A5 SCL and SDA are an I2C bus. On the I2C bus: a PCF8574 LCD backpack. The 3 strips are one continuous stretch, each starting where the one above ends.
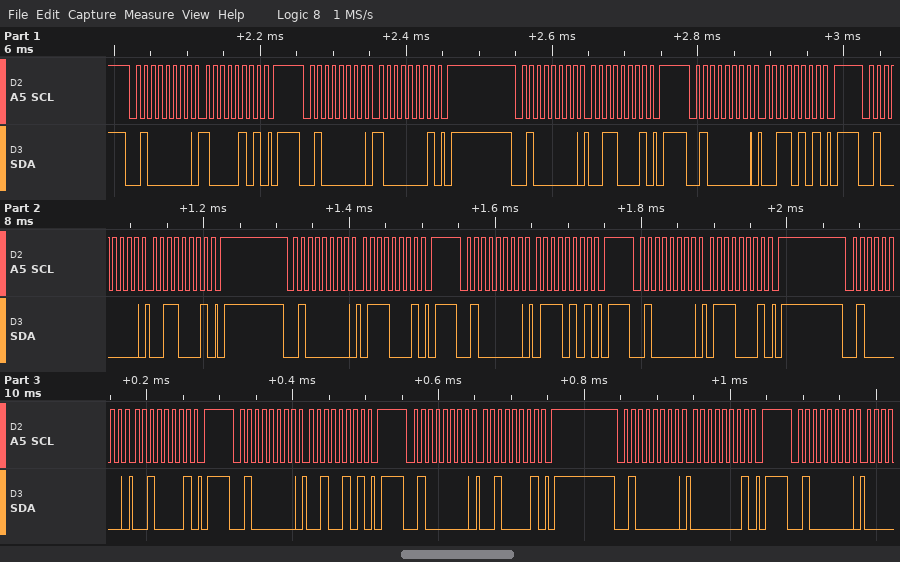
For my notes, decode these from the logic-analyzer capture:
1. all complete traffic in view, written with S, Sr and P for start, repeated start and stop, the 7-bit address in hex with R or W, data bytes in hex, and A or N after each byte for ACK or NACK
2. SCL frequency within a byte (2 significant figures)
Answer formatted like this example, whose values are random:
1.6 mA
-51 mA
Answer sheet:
S 20W A 85 A P S 20W A 81 A P S 20W A 31 A P S 20W A 35 A P S 20W A 31 A P S 20W A 71 A P S 20W A 75 A P S 20W A 71 A P S 20W A 21 A P S 20W A 25 A P S 20W A 21 A P S 20W A 01 A P S 20W A
100 kHz
